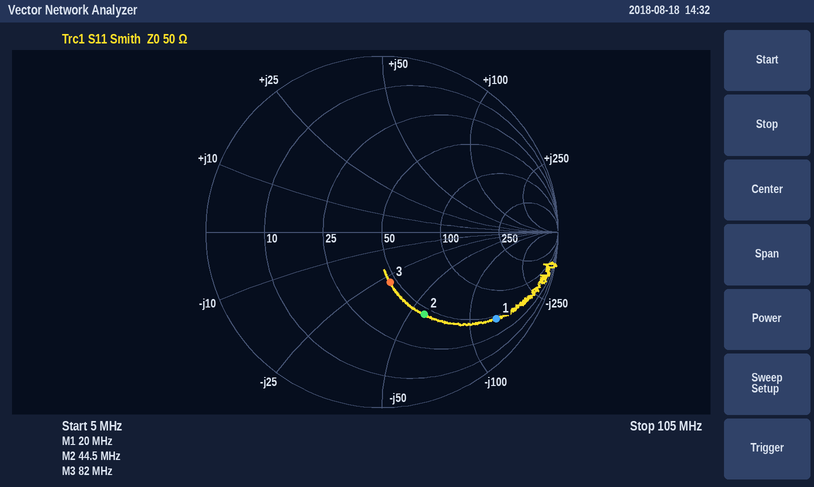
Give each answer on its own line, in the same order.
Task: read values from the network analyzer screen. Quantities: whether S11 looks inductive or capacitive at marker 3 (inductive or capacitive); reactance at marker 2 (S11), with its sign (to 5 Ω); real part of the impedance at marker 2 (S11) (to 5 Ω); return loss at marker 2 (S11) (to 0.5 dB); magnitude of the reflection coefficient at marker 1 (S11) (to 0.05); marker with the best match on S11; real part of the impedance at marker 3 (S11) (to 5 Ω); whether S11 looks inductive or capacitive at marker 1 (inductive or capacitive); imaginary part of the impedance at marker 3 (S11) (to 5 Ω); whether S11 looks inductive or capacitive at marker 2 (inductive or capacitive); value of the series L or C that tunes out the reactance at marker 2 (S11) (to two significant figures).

capacitive
-60 Ω
45 Ω
5.5 dB
0.80
marker 3
45 Ω
capacitive
-30 Ω
capacitive
210 nH
